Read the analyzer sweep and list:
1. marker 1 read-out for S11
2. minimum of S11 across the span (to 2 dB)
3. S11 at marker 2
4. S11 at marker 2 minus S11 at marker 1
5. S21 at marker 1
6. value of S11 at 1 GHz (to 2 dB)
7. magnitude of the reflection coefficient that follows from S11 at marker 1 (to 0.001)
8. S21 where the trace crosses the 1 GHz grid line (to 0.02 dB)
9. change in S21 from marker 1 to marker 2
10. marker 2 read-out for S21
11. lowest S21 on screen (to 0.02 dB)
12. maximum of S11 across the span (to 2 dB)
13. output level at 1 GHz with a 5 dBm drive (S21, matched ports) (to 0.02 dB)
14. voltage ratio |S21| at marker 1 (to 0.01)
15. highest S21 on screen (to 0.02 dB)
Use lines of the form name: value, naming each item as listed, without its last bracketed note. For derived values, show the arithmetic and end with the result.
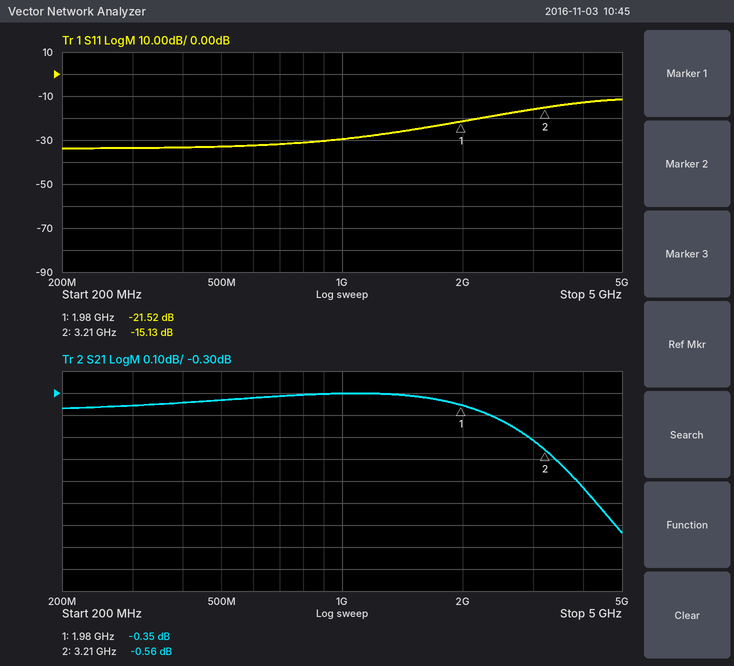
marker 1 read-out for S11: -21.52 dB
minimum of S11 across the span: -34 dB
S11 at marker 2: -15.13 dB
S11 at marker 2 minus S11 at marker 1: -15.13 − (-21.52) = 6.39 dB
S21 at marker 1: -0.35 dB
value of S11 at 1 GHz: -30 dB
magnitude of the reflection coefficient that follows from S11 at marker 1: 10^(-21.52/20) ≈ 0.084
S21 where the trace crosses the 1 GHz grid line: -0.30 dB
change in S21 from marker 1 to marker 2: -0.56 − (-0.35) = -0.21 dB
marker 2 read-out for S21: -0.56 dB
lowest S21 on screen: -0.94 dB
maximum of S11 across the span: -12 dB
output level at 1 GHz with a 5 dBm drive (S21, matched ports): 5 dBm + (-0.30 dB) = 4.70 dBm
voltage ratio |S21| at marker 1: 10^(-0.35/20) ≈ 0.96
highest S21 on screen: -0.30 dB
